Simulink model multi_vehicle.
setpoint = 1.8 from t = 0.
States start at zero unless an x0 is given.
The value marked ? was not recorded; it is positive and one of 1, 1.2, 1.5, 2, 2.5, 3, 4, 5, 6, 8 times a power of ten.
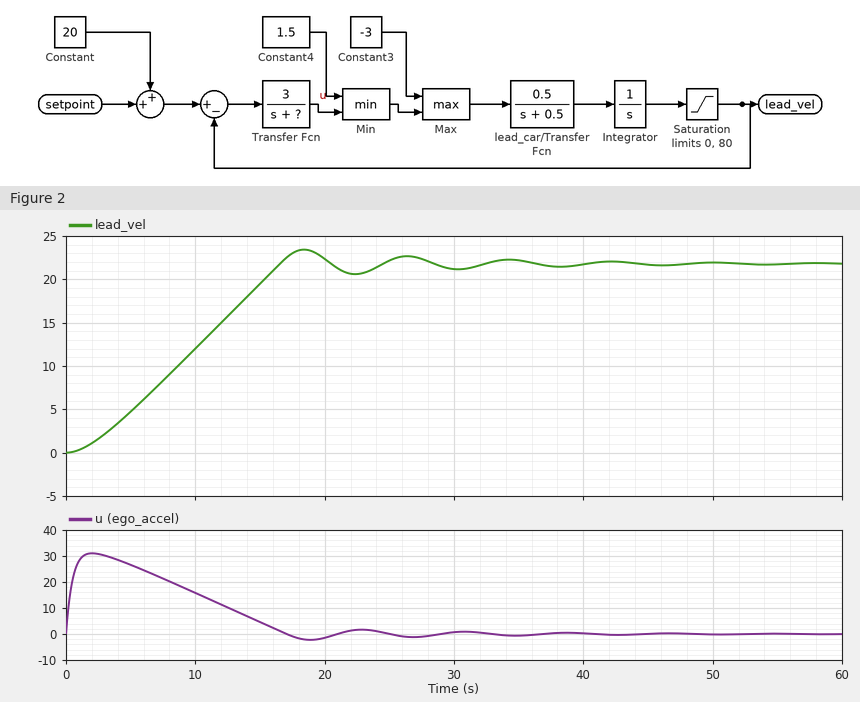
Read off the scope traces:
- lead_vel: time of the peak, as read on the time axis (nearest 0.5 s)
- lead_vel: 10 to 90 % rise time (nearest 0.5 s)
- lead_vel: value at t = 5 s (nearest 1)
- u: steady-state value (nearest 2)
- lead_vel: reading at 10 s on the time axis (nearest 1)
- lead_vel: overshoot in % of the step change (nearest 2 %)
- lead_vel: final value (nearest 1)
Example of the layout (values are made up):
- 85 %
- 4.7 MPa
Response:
- 18.5 s
- 12.0 s
- 5
- 0
- 12
- 8 %
- 22
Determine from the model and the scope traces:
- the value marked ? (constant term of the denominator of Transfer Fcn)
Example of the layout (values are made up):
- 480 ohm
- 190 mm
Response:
- 2
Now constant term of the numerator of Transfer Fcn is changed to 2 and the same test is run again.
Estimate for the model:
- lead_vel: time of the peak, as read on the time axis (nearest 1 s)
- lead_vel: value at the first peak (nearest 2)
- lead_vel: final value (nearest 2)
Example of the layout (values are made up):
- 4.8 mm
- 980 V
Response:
- 19 s
- 24
- 22
